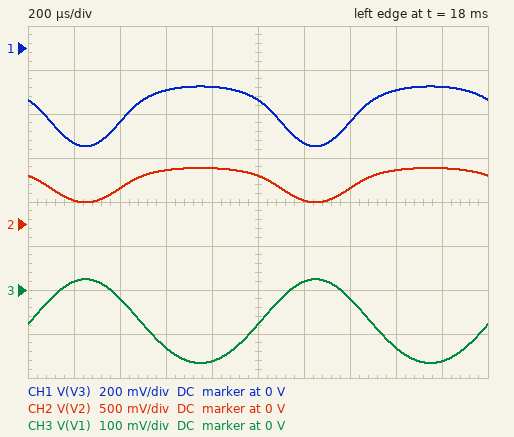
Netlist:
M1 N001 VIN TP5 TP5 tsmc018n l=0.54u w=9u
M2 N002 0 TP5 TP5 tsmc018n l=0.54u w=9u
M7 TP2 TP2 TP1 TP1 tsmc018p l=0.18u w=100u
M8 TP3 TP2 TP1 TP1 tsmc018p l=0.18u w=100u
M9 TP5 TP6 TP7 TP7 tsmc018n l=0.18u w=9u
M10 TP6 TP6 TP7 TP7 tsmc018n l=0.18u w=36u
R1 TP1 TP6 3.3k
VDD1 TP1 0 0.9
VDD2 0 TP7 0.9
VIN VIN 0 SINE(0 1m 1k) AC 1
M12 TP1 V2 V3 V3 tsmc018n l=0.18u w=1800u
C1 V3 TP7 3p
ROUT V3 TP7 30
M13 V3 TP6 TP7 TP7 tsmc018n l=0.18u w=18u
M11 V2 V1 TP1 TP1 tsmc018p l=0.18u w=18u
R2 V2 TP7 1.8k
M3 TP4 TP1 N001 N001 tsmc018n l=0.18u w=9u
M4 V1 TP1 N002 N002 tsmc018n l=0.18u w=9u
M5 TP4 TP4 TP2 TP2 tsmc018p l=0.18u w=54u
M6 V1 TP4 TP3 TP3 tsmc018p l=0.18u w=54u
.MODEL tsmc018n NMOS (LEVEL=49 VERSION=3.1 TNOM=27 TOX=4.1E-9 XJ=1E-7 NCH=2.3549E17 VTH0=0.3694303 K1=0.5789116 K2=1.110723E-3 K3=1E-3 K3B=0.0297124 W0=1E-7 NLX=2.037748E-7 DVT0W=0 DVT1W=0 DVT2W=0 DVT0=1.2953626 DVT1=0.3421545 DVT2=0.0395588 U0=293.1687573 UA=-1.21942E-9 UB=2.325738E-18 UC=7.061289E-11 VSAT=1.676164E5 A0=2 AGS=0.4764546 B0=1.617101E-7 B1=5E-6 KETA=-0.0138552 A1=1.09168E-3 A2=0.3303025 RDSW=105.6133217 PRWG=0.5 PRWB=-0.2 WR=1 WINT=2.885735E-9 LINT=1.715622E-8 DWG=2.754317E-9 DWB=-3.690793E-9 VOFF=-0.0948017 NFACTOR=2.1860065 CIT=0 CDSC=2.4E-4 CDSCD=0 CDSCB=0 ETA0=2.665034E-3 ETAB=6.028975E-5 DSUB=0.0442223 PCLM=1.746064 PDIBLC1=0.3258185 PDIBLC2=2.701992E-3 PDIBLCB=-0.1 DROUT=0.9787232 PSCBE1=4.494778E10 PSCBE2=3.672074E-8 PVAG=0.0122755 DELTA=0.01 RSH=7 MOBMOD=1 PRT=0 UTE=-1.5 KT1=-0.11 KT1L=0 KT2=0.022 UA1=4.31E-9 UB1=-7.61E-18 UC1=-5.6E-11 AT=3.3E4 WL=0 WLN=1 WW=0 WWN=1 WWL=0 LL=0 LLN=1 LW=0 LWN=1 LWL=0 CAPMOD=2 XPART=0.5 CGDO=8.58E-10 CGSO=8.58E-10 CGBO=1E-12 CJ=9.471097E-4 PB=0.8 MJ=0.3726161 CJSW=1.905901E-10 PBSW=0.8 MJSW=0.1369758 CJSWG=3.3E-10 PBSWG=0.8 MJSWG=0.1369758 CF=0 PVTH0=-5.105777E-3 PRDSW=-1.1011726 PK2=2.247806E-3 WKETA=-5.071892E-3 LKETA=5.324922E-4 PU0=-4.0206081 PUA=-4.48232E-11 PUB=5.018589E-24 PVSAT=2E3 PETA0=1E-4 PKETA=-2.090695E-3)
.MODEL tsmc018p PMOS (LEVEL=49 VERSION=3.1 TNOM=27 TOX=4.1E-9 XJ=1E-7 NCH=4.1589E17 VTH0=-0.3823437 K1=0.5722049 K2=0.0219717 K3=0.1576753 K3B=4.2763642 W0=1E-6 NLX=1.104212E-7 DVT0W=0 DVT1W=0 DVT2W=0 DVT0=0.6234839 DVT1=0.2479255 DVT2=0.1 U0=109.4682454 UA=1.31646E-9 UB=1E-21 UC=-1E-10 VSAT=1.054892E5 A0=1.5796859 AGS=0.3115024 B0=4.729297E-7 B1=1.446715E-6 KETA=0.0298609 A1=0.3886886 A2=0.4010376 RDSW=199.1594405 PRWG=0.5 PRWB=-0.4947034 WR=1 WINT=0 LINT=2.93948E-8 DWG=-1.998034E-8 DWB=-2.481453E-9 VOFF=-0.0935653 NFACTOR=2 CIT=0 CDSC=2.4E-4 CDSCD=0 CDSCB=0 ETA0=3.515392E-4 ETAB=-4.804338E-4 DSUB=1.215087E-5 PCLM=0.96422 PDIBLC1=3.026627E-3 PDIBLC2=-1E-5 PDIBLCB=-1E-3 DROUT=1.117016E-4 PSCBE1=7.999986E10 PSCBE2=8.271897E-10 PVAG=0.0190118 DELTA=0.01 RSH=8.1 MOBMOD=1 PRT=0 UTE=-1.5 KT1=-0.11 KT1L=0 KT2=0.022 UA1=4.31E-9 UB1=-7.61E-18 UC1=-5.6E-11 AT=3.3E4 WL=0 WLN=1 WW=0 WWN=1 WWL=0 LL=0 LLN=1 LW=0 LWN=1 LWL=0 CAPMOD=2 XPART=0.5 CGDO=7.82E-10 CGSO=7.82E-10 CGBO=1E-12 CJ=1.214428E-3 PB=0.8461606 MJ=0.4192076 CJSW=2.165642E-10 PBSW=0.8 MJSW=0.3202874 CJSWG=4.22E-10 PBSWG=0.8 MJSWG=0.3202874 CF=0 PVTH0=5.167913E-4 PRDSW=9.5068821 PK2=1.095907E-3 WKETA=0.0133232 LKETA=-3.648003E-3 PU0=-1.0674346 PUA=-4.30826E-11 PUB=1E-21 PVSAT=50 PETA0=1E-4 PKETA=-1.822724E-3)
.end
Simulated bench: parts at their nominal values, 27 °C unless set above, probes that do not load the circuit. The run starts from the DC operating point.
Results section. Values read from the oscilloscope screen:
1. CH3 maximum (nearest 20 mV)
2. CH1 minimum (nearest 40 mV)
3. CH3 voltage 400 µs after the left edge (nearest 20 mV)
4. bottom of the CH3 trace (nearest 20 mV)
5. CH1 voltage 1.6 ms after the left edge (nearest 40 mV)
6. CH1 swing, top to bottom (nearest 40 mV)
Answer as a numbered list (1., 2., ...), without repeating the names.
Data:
1. 20 mV
2. -440 mV
3. -20 mV
4. -160 mV
5. -200 mV
6. 280 mV
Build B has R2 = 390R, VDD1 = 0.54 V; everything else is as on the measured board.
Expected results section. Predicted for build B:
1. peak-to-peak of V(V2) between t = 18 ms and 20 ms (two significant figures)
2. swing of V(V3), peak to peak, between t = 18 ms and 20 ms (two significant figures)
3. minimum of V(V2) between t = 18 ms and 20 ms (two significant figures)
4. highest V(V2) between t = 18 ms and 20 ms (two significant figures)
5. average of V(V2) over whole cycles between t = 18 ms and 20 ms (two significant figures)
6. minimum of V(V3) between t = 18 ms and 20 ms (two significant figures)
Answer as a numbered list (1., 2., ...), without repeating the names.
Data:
1. 41 mV
2. 3.5 mV
3. -580 mV
4. -540 mV
5. -560 mV
6. -900 mV
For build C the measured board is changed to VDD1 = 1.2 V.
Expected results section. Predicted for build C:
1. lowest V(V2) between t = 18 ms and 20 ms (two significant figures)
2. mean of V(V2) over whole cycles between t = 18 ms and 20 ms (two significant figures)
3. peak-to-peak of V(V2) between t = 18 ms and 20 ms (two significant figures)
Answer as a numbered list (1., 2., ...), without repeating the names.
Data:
1. 270 mV
2. 660 mV
3. 630 mV
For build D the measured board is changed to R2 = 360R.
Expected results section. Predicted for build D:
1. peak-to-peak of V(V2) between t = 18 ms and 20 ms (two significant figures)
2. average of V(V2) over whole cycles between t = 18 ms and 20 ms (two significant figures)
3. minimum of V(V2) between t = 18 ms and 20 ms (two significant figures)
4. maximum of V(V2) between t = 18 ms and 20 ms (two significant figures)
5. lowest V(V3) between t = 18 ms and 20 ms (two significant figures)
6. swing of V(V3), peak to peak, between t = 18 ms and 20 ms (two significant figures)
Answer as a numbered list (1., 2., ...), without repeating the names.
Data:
1. 220 mV
2. -540 mV
3. -650 mV
4. -430 mV
5. -900 mV
6. 34 mV
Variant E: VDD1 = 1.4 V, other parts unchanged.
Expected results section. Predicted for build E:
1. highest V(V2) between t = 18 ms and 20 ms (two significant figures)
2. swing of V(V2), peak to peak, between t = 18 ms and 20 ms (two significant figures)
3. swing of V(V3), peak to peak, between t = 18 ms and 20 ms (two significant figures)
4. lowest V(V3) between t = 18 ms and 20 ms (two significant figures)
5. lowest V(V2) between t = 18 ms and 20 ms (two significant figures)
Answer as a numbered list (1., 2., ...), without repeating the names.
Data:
1. 1.1 V
2. 770 mV
3. 540 mV
4. -400 mV
5. 310 mV
